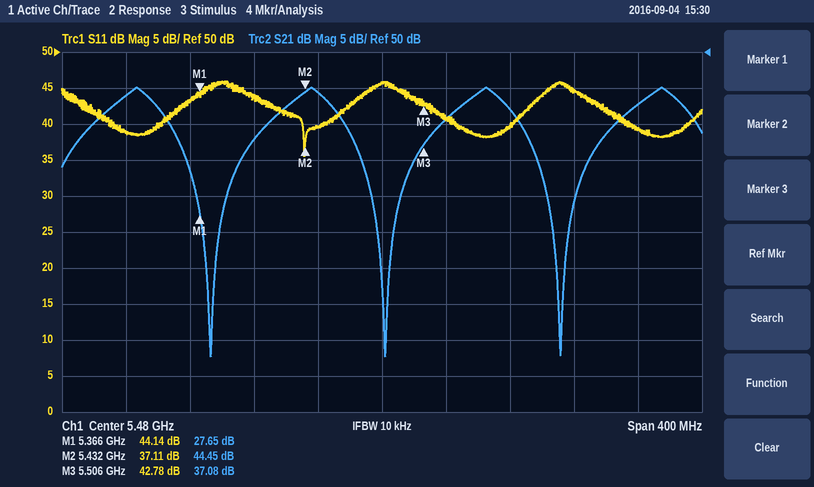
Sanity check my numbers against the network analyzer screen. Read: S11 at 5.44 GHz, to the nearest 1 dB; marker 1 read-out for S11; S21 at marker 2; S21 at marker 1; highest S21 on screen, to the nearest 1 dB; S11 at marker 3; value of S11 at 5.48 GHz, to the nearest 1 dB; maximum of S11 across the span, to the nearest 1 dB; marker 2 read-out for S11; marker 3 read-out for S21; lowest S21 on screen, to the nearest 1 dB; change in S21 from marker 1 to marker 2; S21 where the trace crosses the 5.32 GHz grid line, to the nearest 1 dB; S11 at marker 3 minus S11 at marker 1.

40 dB
44.14 dB
44.45 dB
27.65 dB
45 dB
42.78 dB
46 dB
46 dB
37.11 dB
37.08 dB
8 dB
16.80 dB
44 dB
-1.36 dB
